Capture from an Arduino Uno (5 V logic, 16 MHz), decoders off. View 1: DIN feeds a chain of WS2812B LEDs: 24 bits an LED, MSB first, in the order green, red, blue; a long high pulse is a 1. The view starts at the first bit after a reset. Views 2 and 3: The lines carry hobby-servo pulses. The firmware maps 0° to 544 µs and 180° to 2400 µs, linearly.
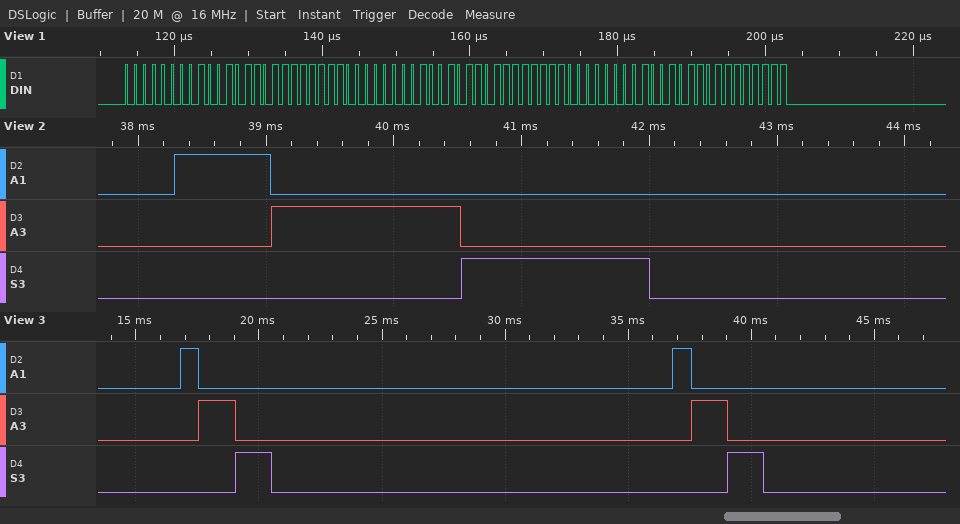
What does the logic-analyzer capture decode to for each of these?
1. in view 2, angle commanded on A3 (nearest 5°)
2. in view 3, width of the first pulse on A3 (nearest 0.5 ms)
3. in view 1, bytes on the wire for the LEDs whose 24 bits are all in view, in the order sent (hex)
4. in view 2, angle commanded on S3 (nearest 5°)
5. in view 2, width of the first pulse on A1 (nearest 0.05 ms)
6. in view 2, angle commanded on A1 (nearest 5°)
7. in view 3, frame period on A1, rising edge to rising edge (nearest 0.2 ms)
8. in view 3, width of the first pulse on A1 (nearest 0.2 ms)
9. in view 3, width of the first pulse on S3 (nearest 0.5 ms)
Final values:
90°
1.5 ms
00 96 FF 00 96 FF 00 96 FF
90°
0.75 ms
20°
20.0 ms
0.8 ms
1.5 ms
